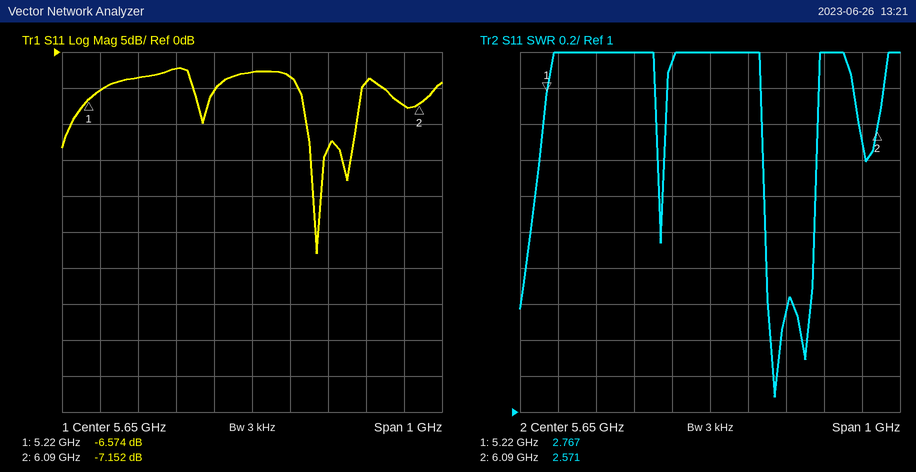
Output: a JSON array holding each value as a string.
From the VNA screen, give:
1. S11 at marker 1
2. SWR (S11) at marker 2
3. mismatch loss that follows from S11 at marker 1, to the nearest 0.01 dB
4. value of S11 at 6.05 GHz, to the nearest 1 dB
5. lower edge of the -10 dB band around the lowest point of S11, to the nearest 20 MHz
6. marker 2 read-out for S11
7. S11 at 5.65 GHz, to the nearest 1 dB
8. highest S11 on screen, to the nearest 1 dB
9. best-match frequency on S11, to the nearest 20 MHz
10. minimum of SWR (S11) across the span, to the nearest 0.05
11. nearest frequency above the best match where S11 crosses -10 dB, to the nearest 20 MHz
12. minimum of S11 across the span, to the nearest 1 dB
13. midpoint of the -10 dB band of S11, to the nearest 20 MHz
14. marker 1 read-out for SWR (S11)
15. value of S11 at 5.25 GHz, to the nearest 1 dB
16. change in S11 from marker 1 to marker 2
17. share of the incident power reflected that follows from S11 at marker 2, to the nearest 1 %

["-6.574 dB", "2.571", "1.08 dB", "-7 dB", "5.80 GHz", "-7.152 dB", "-3 dB", "-2 dB", "5.82 GHz", "1.10", "5.92 GHz", "-28 dB", "5.86 GHz", "2.767", "-5 dB", "-0.578 dB", "19 %"]
